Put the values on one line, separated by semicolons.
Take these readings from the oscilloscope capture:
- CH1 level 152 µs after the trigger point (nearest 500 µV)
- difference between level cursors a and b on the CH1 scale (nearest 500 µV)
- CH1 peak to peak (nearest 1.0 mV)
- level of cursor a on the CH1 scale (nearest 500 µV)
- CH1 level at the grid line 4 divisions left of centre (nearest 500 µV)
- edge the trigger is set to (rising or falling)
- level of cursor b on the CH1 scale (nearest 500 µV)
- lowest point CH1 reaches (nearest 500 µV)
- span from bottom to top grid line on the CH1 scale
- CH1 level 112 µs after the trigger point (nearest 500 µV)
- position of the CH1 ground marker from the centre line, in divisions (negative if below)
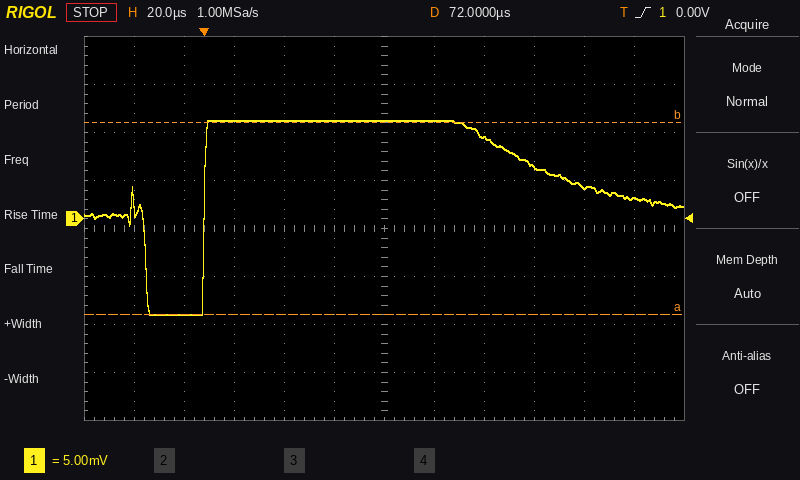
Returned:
3.5 mV; 20.0 mV; 20.0 mV; -10.0 mV; -10.0 mV; rising; 10.0 mV; -10.0 mV; 40 mV; 8.5 mV; +0.2 div
